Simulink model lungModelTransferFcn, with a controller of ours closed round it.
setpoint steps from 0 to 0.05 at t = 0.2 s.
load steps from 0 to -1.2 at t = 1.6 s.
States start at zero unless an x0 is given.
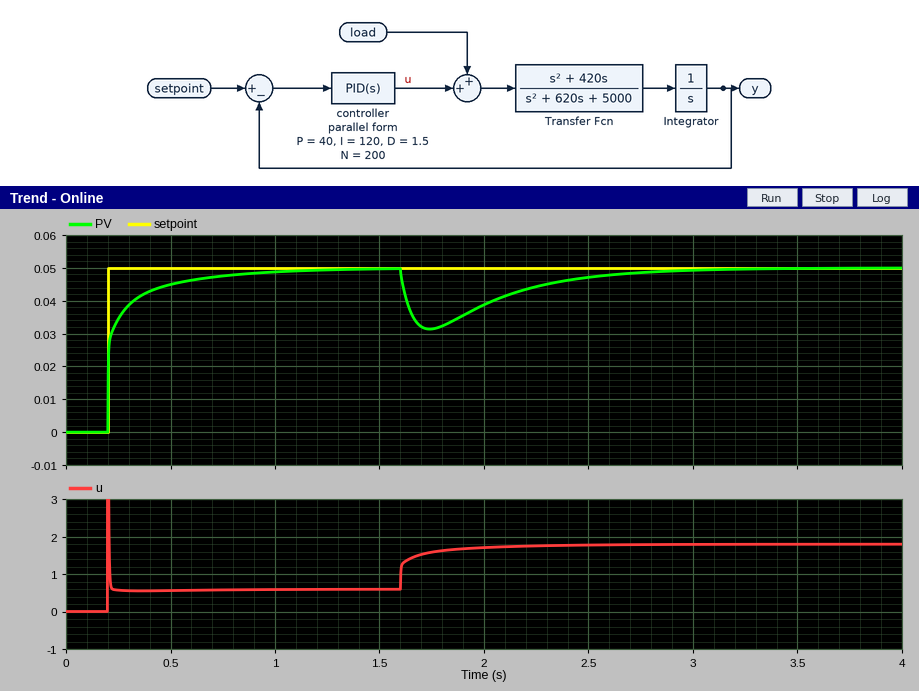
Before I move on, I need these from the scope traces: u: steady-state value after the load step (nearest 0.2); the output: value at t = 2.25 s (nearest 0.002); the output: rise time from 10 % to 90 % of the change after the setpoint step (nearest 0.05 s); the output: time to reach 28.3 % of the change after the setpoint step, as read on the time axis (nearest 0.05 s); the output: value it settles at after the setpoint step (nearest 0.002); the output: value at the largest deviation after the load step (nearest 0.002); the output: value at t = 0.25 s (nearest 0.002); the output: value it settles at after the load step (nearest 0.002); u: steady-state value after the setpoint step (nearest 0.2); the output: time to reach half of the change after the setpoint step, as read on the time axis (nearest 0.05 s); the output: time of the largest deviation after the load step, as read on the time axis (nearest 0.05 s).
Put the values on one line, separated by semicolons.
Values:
1.8; 0.044; 0.30 s; 0.20 s; 0.050; 0.032; 0.034; 0.050; 0.6; 0.20 s; 1.75 s
